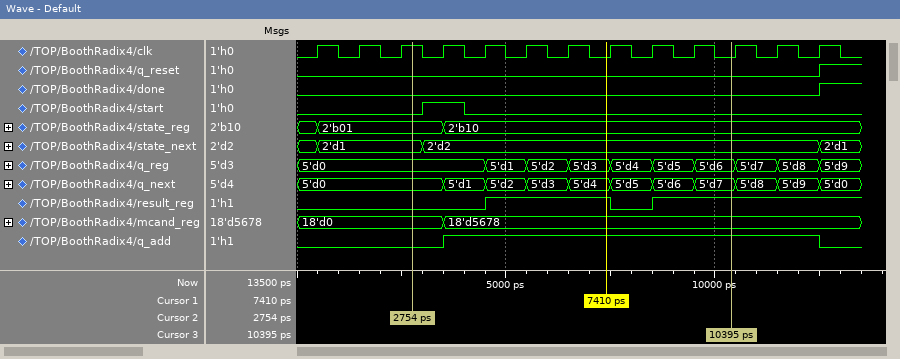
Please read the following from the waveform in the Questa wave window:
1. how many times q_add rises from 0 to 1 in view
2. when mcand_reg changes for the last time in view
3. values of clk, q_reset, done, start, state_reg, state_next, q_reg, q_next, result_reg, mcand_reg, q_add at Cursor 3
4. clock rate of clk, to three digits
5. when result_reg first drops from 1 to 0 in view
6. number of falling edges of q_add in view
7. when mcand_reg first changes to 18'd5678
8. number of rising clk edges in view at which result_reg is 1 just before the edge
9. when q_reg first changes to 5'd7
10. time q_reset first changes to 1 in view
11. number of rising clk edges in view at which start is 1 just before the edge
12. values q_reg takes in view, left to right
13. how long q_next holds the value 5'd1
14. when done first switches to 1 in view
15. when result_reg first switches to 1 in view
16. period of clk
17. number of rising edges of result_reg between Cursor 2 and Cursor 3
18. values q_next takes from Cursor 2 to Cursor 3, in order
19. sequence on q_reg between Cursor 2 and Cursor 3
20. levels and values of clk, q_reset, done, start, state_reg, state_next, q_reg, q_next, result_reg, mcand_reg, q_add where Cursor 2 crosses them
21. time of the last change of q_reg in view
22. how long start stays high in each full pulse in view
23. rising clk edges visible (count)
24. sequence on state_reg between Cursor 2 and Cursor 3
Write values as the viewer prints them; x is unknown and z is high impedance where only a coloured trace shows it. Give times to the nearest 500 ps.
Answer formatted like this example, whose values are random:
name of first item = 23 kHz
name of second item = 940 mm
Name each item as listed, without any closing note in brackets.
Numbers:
how many times q_add rises from 0 to 1 in view = 1
when mcand_reg changes for the last time in view = 3500 ps
values of clk, q_reset, done, start, state_reg, state_next, q_reg, q_next, result_reg, mcand_reg, q_add at Cursor 3 = clk=0, q_reset=0, done=0, start=0, state_reg=2'b10, state_next=2'd2, q_reg=5'd6, q_next=5'd7, result_reg=1, mcand_reg=18'd5678, q_add=1
clock rate of clk, to three digits = 1.00 GHz
when result_reg first drops from 1 to 0 in view = 7500 ps
number of falling edges of q_add in view = 1
when mcand_reg first changes to 18'd5678 = 3500 ps
number of rising clk edges in view at which result_reg is 1 just before the edge = 7
when q_reg first changes to 5'd7 = 10500 ps
time q_reset first changes to 1 in view = 12500 ps
number of rising clk edges in view at which start is 1 just before the edge = 1
values q_reg takes in view, left to right = 5'd0, 5'd1, 5'd2, 5'd3, 5'd4, 5'd5, 5'd6, 5'd7, 5'd8, 5'd9
how long q_next holds the value 5'd1 = 1000 ps
when done first switches to 1 in view = 12500 ps
when result_reg first switches to 1 in view = 4500 ps
period of clk = 1000 ps
number of rising edges of result_reg between Cursor 2 and Cursor 3 = 2
values q_next takes from Cursor 2 to Cursor 3, in order = 5'd0, 5'd1, 5'd2, 5'd3, 5'd4, 5'd5, 5'd6, 5'd7
sequence on q_reg between Cursor 2 and Cursor 3 = 5'd0, 5'd1, 5'd2, 5'd3, 5'd4, 5'd5, 5'd6
levels and values of clk, q_reset, done, start, state_reg, state_next, q_reg, q_next, result_reg, mcand_reg, q_add where Cursor 2 crosses them = clk=1, q_reset=0, done=0, start=0, state_reg=2'b01, state_next=2'd1, q_reg=5'd0, q_next=5'd0, result_reg=0, mcand_reg=18'd0, q_add=0
time of the last change of q_reg in view = 12500 ps
how long start stays high in each full pulse in view = 1000 ps
rising clk edges visible = 13
sequence on state_reg between Cursor 2 and Cursor 3 = 2'b01, 2'b10
